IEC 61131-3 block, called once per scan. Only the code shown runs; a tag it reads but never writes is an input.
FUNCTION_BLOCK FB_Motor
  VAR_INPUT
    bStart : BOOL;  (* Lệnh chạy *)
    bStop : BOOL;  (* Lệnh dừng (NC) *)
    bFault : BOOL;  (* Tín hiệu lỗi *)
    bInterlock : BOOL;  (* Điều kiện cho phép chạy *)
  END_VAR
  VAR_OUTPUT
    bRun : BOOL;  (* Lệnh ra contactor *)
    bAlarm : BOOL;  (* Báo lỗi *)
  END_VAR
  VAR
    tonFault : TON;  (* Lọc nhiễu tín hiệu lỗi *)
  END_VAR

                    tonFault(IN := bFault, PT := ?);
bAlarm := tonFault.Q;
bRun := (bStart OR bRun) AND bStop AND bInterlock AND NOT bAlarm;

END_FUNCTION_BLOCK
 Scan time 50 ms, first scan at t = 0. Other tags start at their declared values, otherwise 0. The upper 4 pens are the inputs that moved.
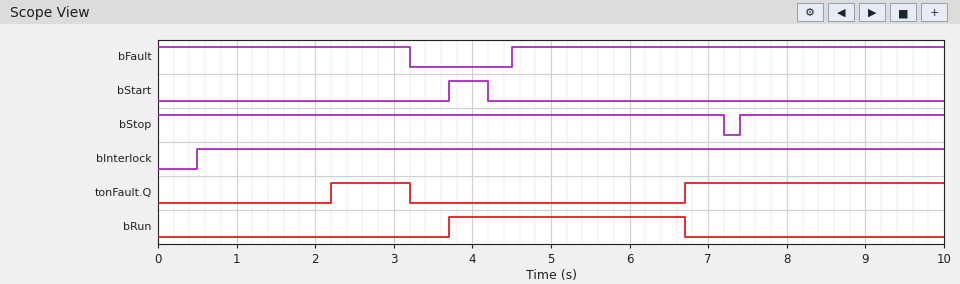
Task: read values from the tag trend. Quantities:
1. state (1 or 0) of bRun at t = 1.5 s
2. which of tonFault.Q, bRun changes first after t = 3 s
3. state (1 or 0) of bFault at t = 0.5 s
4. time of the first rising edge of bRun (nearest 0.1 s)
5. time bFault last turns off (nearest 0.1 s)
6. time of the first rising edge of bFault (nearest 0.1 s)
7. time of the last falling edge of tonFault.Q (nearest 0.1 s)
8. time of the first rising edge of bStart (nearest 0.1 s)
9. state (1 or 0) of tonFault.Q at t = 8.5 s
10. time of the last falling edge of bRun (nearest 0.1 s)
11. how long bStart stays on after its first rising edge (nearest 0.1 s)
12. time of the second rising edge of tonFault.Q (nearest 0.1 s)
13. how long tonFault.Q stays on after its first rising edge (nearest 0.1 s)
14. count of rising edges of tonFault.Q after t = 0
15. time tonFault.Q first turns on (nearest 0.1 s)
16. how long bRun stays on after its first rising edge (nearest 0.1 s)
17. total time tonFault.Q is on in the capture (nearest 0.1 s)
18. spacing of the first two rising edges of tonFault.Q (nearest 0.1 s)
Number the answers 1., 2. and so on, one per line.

1. 0
2. tonFault.Q
3. 1
4. 3.7 s
5. 3.2 s
6. 4.5 s
7. 3.2 s
8. 3.7 s
9. 1
10. 6.7 s
11. 0.5 s
12. 6.7 s
13. 1.0 s
14. 2
15. 2.2 s
16. 3.0 s
17. 4.3 s
18. 4.5 s
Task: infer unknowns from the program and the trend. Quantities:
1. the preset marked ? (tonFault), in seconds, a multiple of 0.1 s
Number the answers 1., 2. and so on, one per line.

1. 2.2 s
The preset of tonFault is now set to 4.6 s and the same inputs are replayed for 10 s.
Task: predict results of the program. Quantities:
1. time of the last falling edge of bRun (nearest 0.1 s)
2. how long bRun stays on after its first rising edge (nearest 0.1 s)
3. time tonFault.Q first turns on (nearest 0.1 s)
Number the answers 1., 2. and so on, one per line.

1. 7.2 s
2. 3.5 s
3. 9.1 s
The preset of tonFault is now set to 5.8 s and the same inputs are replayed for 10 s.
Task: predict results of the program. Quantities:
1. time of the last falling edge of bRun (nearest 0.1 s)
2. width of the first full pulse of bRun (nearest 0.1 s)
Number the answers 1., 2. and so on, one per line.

1. 7.2 s
2. 3.5 s
